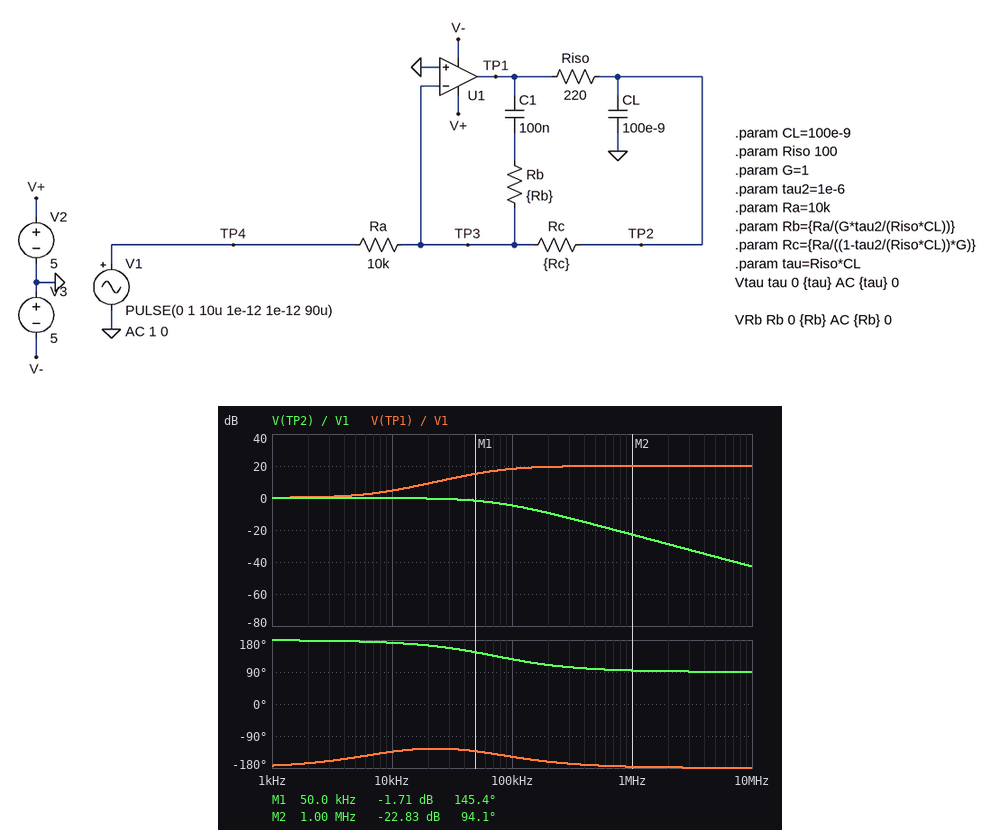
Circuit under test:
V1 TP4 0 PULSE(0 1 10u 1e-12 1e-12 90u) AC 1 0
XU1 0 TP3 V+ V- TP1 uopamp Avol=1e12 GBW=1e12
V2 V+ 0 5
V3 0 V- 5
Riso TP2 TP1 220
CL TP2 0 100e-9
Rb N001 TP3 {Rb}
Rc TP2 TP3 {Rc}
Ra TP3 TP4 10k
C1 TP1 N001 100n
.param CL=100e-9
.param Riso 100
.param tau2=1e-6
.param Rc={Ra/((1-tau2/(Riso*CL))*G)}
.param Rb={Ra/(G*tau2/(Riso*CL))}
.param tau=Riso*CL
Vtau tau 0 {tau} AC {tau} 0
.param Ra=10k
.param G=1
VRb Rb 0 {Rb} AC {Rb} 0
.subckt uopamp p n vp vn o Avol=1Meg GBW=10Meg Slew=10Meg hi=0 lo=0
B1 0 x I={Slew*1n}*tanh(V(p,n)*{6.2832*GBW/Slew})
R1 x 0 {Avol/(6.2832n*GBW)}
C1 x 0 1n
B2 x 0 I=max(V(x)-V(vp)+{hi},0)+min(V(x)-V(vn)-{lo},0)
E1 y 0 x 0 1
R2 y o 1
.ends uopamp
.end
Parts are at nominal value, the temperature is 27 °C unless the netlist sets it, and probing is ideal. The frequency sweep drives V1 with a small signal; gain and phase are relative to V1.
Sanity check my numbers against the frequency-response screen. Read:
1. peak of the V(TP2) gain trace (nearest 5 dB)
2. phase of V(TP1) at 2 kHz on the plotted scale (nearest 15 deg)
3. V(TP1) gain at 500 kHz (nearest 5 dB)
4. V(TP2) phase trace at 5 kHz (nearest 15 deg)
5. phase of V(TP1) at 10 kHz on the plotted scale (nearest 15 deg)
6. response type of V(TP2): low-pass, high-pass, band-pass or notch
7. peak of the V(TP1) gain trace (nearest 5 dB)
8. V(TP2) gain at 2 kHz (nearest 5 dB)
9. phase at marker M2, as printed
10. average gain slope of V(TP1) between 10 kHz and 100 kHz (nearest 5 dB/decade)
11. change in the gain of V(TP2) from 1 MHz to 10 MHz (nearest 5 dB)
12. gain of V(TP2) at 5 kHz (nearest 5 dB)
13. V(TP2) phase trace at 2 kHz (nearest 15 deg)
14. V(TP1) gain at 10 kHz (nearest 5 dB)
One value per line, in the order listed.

0 dB
-165 deg
20 dB
180 deg
-135 deg
low-pass
20 dB
0 dB
94.1 deg
15 dB/decade
-20 dB
0 dB
180 deg
5 dB
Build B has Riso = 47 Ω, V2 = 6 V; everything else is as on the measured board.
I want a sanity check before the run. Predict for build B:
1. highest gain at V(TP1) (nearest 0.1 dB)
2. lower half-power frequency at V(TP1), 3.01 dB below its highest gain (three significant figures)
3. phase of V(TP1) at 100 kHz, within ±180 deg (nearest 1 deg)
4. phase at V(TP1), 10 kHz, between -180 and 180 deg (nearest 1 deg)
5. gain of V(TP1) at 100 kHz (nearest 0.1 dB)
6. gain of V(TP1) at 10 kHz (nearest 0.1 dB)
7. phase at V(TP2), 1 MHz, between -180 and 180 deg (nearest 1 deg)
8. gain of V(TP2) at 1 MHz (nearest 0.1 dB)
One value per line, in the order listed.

20.0 dB
335 kHz
-125 deg
-165 deg
9.5 dB
0.4 dB
109 deg
-9.9 dB
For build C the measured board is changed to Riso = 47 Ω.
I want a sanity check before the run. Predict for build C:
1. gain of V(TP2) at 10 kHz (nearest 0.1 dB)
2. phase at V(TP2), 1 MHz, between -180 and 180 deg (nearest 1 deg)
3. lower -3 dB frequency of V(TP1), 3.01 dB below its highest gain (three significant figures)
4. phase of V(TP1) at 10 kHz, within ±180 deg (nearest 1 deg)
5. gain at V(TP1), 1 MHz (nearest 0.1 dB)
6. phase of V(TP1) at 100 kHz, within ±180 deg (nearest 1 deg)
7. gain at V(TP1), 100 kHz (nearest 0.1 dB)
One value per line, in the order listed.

0 dB
109 deg
335 kHz
-165 deg
19.5 dB
-125 deg
9.5 dB
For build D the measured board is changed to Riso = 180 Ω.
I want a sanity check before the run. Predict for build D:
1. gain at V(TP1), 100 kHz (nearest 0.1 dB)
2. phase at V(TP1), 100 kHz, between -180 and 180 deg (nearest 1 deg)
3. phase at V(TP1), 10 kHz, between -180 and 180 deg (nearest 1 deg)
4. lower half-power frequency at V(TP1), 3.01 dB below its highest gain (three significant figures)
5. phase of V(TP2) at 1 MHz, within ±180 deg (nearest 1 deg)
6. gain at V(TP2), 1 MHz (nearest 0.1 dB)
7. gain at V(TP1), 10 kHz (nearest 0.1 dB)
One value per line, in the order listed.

17.5 dB
-144 deg
-138 deg
87.6 kHz
95 deg
-21.1 dB
3.6 dB
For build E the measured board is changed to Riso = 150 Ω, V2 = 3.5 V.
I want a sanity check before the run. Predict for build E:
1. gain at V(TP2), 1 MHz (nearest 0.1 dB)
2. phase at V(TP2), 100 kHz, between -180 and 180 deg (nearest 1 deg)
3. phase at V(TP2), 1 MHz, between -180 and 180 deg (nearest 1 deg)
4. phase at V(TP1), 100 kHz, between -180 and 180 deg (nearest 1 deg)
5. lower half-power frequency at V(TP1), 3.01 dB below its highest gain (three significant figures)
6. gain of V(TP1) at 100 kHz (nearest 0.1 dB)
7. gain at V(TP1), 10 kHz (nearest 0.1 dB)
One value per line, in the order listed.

-19.5 dB
137 deg
96 deg
-139 deg
105 kHz
16.8 dB
2.8 dB
